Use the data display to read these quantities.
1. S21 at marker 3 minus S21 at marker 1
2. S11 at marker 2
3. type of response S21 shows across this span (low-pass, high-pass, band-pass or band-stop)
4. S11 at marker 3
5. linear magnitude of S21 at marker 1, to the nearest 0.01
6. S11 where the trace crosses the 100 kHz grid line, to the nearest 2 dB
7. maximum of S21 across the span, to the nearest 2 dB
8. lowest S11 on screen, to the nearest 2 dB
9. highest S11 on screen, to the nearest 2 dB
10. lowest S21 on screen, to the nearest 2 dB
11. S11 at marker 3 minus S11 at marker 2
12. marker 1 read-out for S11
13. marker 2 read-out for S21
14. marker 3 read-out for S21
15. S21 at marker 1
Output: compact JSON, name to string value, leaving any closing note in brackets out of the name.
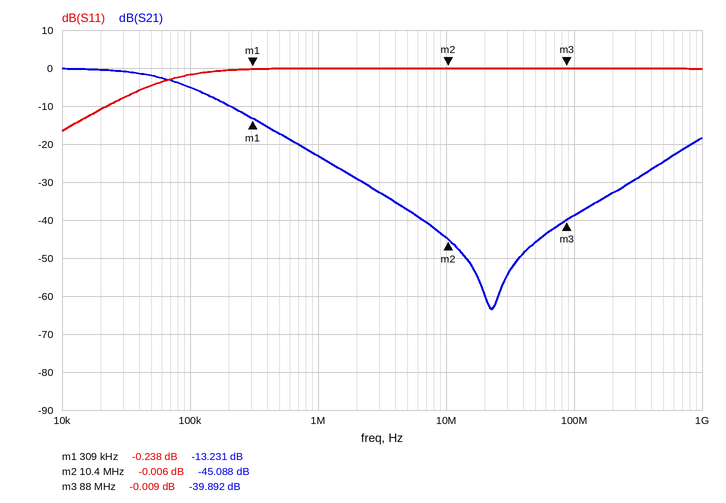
{"S21 at marker 3 minus S21 at marker 1": "-26.661 dB", "S11 at marker 2": "-0.006 dB", "type of response S21 shows across this span": "low-pass", "S11 at marker 3": "-0.009 dB", "linear magnitude of S21 at marker 1, to the nearest 0.01": "0.22", "S11 where the trace crosses the 100 kHz grid line, to the nearest 2 dB": "-2 dB", "maximum of S21 across the span, to the nearest 2 dB": "0 dB", "lowest S11 on screen, to the nearest 2 dB": "-16 dB", "highest S11 on screen, to the nearest 2 dB": "0 dB", "lowest S21 on screen, to the nearest 2 dB": "-64 dB", "S11 at marker 3 minus S11 at marker 2": "-0.003 dB", "marker 1 read-out for S11": "-0.238 dB", "marker 2 read-out for S21": "-45.088 dB", "marker 3 read-out for S21": "-39.892 dB", "S21 at marker 1": "-13.231 dB"}
